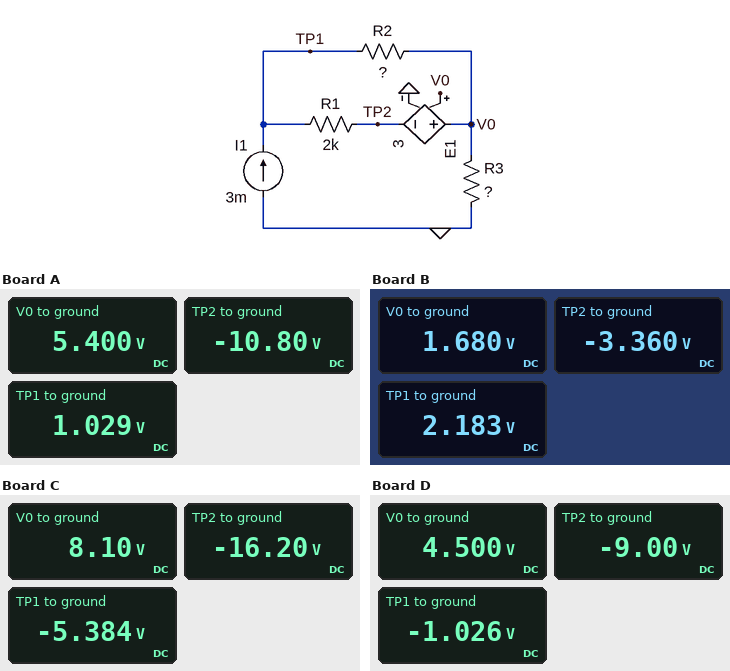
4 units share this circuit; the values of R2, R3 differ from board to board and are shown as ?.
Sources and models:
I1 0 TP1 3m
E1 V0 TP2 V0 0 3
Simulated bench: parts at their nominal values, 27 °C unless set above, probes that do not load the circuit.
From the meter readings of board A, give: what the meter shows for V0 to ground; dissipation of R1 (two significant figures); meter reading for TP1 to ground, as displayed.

5.400 V
70 mW
1.029 V
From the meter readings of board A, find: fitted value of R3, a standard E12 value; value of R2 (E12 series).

1.8 kΩ
1.5 kΩ
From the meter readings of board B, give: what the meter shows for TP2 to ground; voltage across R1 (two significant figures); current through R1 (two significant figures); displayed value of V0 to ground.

-3.360 V
5.5 V
2.8 mA
1.680 V
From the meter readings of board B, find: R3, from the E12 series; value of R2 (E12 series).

560 Ω
2.2 kΩ
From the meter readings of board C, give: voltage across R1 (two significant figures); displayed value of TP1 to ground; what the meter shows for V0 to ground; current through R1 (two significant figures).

11 V
-5.384 V
8.10 V
5.4 mA
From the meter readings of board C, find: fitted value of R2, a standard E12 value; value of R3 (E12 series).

5.6 kΩ
2.7 kΩ
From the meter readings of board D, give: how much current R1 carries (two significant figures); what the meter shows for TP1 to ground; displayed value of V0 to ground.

4.0 mA
-1.026 V
4.500 V
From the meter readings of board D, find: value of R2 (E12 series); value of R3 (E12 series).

5.6 kΩ
1.5 kΩ
